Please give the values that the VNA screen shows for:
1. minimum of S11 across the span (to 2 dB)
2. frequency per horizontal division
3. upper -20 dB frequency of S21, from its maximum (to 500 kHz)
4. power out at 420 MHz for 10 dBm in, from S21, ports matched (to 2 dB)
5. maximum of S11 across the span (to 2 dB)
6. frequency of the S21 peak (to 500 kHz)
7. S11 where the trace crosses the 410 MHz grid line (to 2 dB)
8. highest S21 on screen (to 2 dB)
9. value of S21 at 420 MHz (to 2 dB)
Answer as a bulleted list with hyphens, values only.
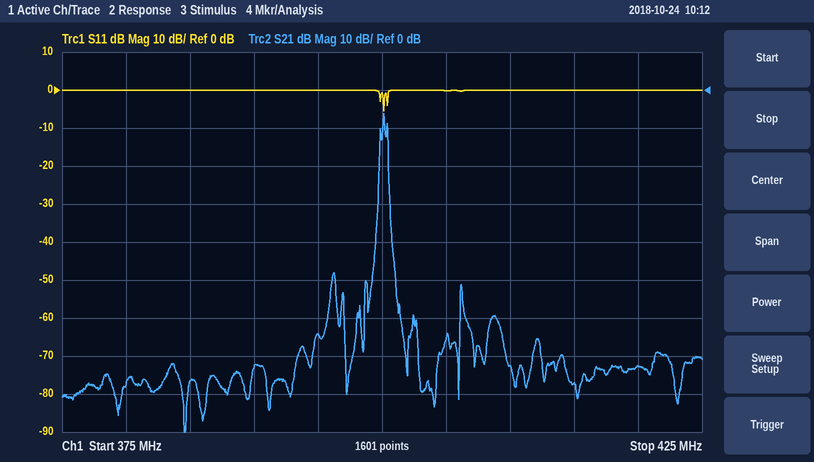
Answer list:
- -6 dB
- 5 MHz
- 400.5 MHz
- -62 dBm
- 0 dB
- 400.0 MHz
- 0 dB
- -6 dB
- -72 dB
